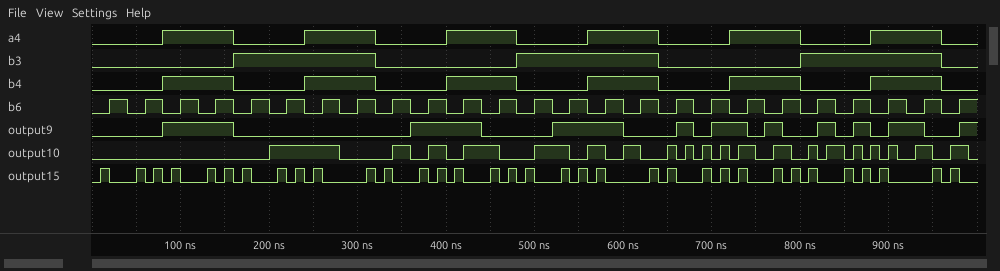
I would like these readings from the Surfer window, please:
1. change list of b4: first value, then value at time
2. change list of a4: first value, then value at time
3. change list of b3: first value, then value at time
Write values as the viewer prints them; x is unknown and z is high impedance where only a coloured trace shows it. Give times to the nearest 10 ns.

0, 1 at 80 ns, 0 at 160 ns, 1 at 240 ns, 0 at 320 ns, 1 at 400 ns, 0 at 480 ns, 1 at 560 ns, 0 at 640 ns, 1 at 720 ns, 0 at 800 ns, 1 at 880 ns, 0 at 960 ns
0, 1 at 80 ns, 0 at 160 ns, 1 at 240 ns, 0 at 320 ns, 1 at 400 ns, 0 at 480 ns, 1 at 560 ns, 0 at 640 ns, 1 at 720 ns, 0 at 800 ns, 1 at 880 ns, 0 at 960 ns
0, 1 at 160 ns, 0 at 320 ns, 1 at 480 ns, 0 at 640 ns, 1 at 800 ns, 0 at 960 ns
